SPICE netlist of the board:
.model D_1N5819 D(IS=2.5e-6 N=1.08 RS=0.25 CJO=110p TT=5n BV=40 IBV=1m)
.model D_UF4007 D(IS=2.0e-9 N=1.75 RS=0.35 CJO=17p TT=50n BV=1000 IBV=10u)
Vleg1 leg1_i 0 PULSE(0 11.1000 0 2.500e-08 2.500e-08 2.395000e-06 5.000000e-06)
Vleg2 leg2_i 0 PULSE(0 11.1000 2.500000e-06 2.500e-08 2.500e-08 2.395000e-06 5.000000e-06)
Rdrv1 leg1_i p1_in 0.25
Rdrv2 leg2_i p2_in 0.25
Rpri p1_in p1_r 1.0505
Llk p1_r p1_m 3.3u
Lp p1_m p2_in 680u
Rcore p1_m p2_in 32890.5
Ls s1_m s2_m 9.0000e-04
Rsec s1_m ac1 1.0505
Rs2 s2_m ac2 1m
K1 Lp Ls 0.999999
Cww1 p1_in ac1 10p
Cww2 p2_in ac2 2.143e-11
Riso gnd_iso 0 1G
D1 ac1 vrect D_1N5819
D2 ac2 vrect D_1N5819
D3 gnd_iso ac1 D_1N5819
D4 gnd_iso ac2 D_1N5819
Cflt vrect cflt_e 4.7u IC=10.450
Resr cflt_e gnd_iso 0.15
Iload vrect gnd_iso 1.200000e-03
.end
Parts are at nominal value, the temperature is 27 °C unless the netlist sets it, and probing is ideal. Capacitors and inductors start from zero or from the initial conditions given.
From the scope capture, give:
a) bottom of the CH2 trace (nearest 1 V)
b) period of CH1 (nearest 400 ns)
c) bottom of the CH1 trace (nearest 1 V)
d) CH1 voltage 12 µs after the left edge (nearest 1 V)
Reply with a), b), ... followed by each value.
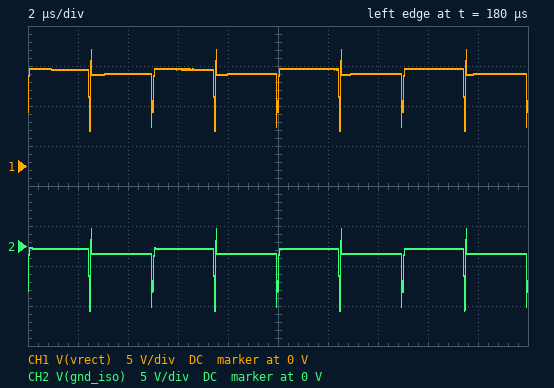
a) -8 V
b) 2.4 µs
c) 4 V
d) 12 V
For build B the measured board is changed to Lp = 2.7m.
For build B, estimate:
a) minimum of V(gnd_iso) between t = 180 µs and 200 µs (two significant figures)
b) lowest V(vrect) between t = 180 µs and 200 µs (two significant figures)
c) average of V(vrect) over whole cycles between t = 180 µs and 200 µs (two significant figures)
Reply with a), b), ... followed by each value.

a) -5.7 V
b) 4.7 V
c) 11 V
